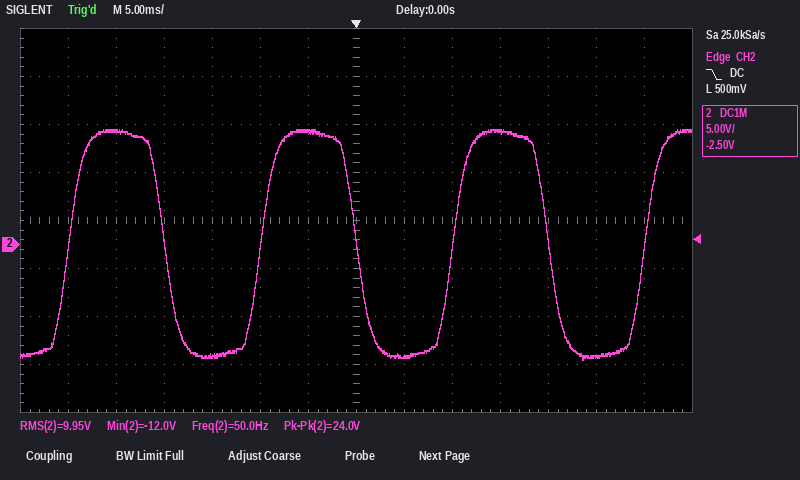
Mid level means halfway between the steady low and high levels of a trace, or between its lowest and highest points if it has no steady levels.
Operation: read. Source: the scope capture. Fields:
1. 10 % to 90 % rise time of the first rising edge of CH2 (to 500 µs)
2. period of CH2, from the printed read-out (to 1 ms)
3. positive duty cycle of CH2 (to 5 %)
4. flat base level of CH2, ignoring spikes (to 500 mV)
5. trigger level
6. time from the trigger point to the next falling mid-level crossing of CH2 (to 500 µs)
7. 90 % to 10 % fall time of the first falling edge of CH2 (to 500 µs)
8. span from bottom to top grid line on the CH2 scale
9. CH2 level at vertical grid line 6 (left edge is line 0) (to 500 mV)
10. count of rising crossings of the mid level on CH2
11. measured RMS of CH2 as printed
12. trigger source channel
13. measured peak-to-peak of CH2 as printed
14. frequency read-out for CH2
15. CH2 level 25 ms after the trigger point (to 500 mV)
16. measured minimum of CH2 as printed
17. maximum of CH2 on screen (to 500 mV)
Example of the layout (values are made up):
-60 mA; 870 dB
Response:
3.0 ms; 20 ms; 50 %; -11.5 V; 500 mV; 20.0 ms; 3.0 ms; 40 V; 12.0 V; 4; 9.95 V; CH2; 24.0 V; 50.0 Hz; -11.5 V; -12.0 V; 12.0 V
